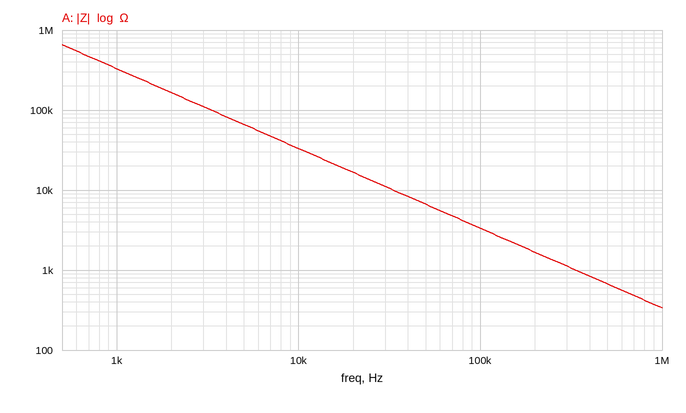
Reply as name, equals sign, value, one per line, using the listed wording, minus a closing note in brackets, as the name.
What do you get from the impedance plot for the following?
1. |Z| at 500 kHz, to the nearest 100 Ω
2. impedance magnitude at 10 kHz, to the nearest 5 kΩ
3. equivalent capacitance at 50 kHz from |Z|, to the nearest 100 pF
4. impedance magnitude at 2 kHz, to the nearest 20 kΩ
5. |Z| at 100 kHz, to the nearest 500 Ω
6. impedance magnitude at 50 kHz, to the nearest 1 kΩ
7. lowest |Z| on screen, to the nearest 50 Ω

|Z| at 500 kHz, to the nearest 100 Ω = 700 Ω
impedance magnitude at 10 kHz, to the nearest 5 kΩ = 35 kΩ
equivalent capacitance at 50 kHz from |Z|, to the nearest 100 pF = 500 pF
impedance magnitude at 2 kHz, to the nearest 20 kΩ = 160 kΩ
|Z| at 100 kHz, to the nearest 500 Ω = 3.5 kΩ
impedance magnitude at 50 kHz, to the nearest 1 kΩ = 7 kΩ
lowest |Z| on screen, to the nearest 50 Ω = 350 Ω
